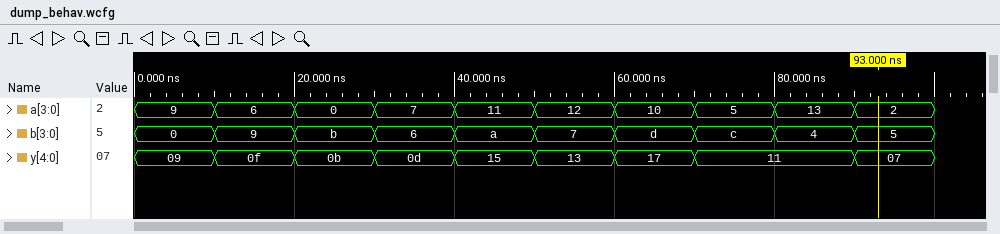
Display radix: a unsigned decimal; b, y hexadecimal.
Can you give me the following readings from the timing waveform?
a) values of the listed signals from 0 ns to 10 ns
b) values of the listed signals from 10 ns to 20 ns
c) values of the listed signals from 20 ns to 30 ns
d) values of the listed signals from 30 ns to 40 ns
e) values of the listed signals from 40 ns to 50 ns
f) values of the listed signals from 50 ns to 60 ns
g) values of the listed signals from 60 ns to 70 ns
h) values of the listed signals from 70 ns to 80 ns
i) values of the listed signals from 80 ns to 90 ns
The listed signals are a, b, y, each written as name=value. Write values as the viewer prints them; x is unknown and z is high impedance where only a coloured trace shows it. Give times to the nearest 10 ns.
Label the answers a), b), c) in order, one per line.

a) a=9, b=0, y=09
b) a=6, b=9, y=0f
c) a=0, b=b, y=0b
d) a=7, b=6, y=0d
e) a=11, b=a, y=15
f) a=12, b=7, y=13
g) a=10, b=d, y=17
h) a=5, b=c, y=11
i) a=13, b=4, y=11
